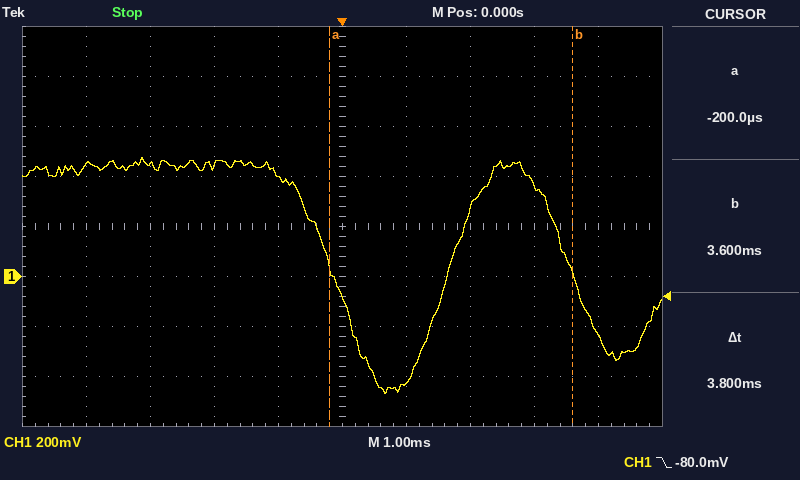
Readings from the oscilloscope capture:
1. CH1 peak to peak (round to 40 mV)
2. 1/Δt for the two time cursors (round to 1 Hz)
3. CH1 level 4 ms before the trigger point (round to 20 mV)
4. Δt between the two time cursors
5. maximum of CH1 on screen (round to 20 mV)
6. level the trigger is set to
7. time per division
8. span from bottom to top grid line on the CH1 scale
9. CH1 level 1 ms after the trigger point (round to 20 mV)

960 mV
263 Hz
440 mV
3.8 ms
480 mV
-80.0 mV
1 ms
1.6 V
-420 mV
